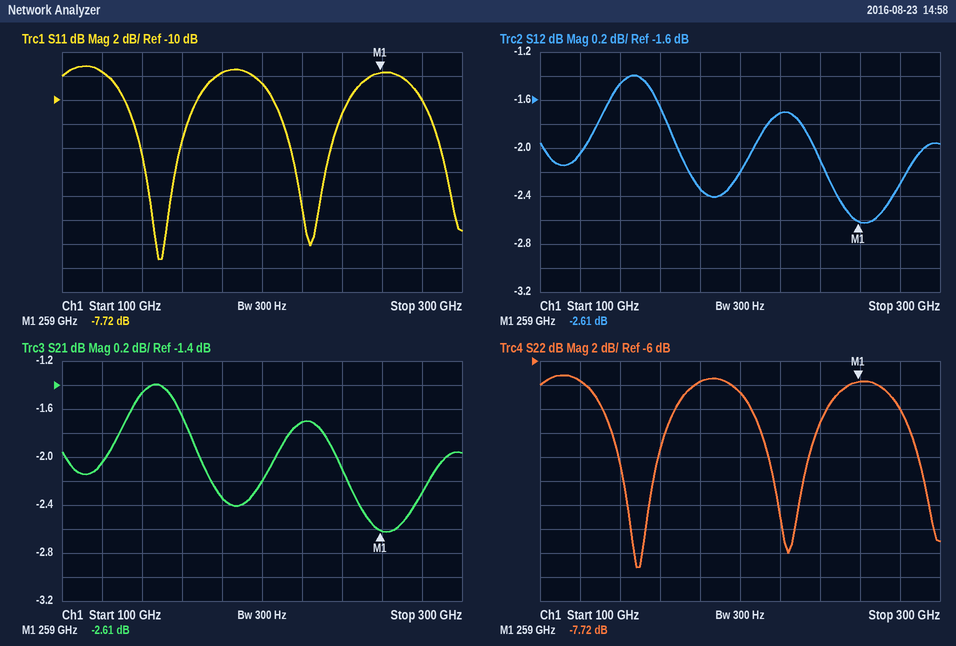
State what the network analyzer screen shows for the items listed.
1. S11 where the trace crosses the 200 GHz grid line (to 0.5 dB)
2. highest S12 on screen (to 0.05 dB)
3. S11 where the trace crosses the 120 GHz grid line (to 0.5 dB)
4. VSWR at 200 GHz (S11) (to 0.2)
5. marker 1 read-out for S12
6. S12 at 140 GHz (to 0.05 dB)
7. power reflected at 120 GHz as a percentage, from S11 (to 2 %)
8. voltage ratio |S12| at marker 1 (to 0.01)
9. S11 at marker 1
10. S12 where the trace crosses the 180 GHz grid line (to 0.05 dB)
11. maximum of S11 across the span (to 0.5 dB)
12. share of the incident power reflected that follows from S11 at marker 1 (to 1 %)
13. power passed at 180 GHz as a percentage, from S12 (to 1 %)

-8.5 dB
-1.40 dB
-7.5 dB
2.2
-2.61 dB
-1.45 dB
18 %
0.74
-7.72 dB
-2.35 dB
-7.0 dB
17 %
58 %
